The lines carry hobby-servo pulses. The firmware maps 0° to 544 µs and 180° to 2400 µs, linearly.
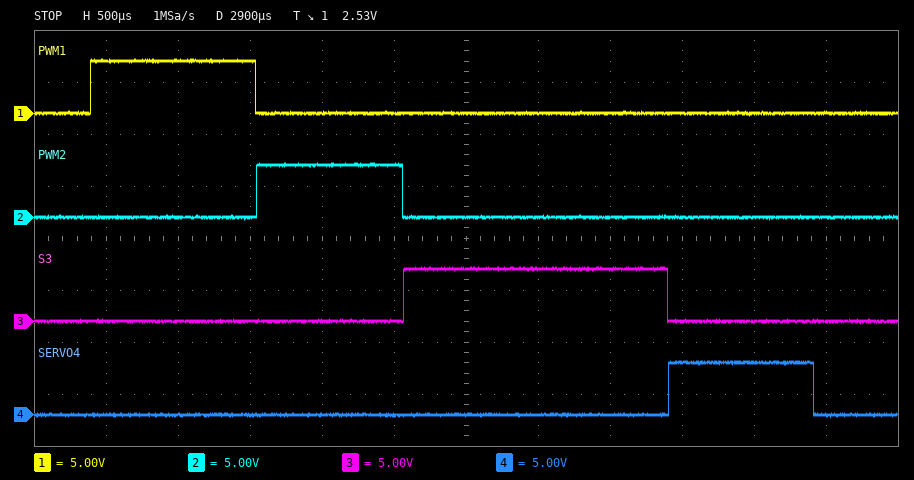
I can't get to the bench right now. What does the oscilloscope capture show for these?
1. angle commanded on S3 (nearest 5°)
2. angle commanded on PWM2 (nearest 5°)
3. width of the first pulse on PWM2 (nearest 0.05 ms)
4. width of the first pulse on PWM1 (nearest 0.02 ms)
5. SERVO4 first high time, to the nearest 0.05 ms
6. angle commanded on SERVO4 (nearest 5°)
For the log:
125°
45°
1.00 ms
1.14 ms
1.00 ms
45°
